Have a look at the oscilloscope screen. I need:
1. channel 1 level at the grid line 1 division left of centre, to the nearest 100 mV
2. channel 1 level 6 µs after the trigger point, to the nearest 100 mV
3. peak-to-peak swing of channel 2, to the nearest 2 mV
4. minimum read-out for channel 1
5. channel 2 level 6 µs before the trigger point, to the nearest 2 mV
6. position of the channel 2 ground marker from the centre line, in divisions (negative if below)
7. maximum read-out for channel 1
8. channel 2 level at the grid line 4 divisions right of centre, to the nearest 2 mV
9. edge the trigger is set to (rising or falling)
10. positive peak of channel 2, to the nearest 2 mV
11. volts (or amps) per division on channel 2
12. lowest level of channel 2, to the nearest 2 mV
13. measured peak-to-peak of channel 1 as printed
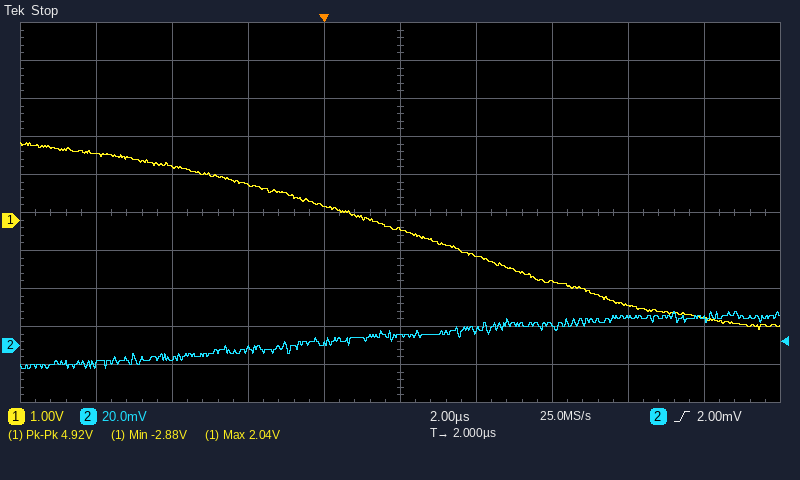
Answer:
400 mV
-1.6 V
30 mV
-2.88 V
-10 mV
-3.5 div
2.04 V
14 mV
rising
18 mV
20 mV
-12 mV
4.92 V
